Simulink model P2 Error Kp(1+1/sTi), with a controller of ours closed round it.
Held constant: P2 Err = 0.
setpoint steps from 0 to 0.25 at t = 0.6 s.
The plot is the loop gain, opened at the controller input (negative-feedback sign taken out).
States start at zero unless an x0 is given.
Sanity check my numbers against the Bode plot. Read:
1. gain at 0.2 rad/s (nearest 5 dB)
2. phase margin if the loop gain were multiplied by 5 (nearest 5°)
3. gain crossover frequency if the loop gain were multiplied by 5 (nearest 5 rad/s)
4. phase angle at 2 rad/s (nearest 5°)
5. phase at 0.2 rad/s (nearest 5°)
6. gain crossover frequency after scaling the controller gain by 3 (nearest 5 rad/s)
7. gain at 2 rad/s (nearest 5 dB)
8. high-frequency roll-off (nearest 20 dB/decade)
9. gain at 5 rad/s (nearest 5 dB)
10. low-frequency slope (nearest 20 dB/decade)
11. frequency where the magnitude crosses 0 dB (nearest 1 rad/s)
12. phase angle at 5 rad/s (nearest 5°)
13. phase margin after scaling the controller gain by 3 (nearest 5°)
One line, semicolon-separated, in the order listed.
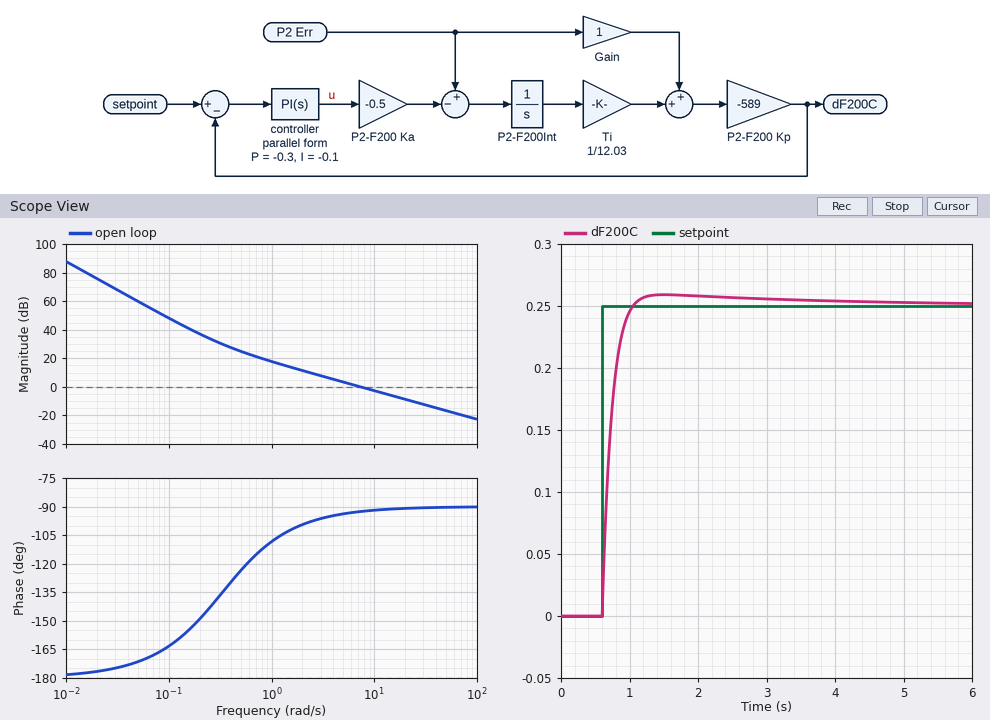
35 dB; 90°; 35 rad/s; -100°; -150°; 20 rad/s; 10 dB; -20 dB/decade; 5 dB; -40 dB/decade; 7 rad/s; -95°; 90°
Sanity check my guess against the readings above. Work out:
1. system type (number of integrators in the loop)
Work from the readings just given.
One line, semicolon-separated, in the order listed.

2
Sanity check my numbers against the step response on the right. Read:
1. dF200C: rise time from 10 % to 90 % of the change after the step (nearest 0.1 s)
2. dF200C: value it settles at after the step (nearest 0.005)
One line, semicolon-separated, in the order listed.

0.3 s; 0.250
